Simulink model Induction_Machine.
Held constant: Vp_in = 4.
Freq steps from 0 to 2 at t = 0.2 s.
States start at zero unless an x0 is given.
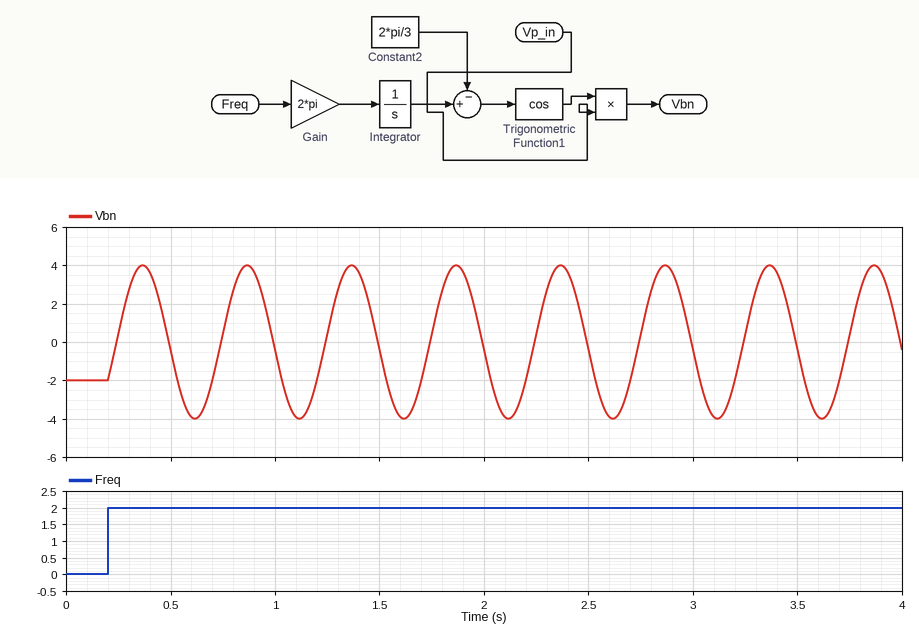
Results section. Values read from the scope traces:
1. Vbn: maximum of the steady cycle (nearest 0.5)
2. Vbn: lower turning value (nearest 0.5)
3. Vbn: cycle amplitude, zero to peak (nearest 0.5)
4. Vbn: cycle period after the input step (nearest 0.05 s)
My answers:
4.0
-4.0
4.0
0.50 s
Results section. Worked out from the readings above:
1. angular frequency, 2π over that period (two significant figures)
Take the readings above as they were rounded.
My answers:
13 rad/s
